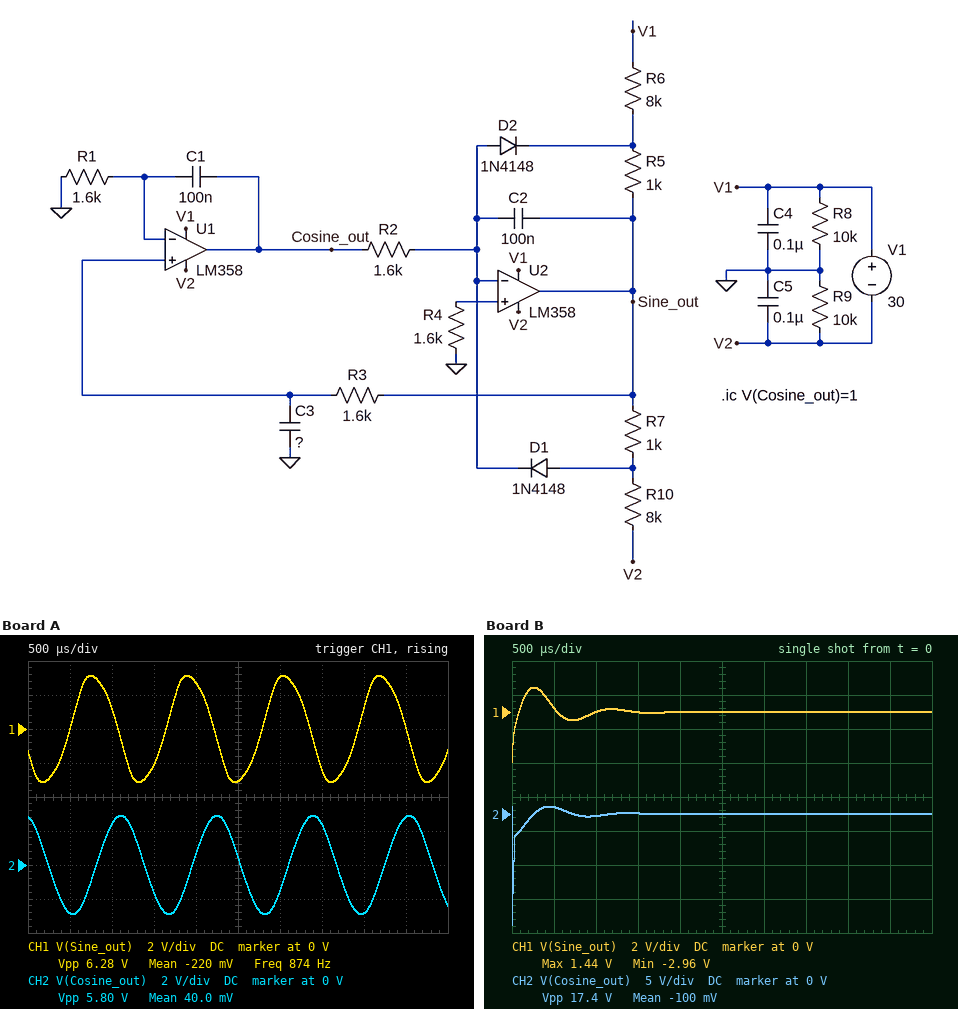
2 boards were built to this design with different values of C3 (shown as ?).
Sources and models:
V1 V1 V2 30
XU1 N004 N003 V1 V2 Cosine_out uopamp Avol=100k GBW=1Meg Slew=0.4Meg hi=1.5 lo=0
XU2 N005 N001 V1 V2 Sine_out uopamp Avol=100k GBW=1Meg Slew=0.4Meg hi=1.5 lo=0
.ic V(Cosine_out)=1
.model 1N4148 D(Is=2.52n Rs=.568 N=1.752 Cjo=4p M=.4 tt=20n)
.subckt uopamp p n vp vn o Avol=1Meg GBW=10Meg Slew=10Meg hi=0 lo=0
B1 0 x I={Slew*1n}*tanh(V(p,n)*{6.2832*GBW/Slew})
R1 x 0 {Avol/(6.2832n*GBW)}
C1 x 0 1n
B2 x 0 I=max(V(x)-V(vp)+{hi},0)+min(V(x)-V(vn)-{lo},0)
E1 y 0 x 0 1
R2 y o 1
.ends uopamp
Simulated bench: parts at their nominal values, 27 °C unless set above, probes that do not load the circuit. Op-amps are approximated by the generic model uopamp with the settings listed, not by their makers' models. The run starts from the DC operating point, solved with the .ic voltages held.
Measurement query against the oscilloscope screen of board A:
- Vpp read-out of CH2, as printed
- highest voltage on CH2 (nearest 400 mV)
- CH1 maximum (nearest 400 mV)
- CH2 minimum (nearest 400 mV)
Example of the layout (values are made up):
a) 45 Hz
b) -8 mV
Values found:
a) 5.80 V
b) 2.8 V
c) 3.2 V
d) -2.8 V
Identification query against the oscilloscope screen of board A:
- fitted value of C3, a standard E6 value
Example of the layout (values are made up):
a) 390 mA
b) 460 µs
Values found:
a) 150 nF
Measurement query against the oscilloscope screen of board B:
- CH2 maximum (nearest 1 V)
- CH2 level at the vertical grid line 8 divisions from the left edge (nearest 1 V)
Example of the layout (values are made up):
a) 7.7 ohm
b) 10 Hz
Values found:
a) 1 V
b) 0 V
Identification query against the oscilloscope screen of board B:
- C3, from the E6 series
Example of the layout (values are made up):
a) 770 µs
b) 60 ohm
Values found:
a) 33 nF
